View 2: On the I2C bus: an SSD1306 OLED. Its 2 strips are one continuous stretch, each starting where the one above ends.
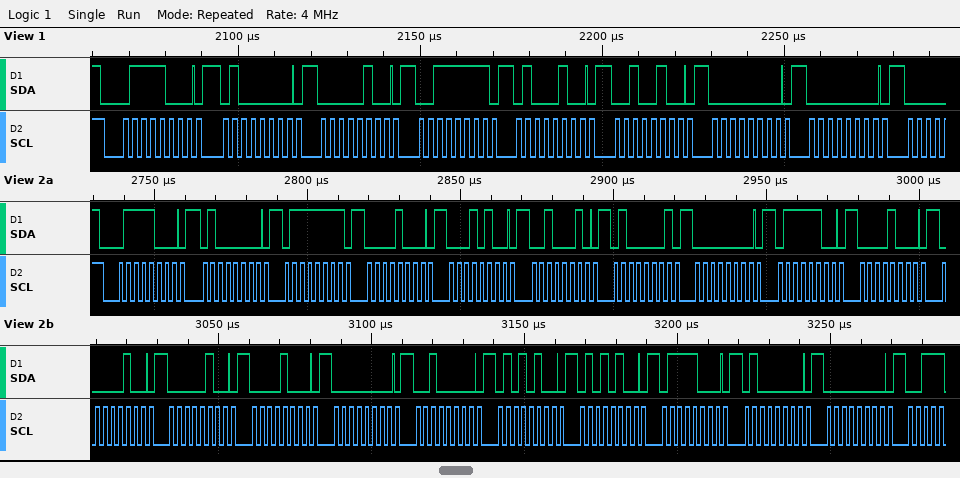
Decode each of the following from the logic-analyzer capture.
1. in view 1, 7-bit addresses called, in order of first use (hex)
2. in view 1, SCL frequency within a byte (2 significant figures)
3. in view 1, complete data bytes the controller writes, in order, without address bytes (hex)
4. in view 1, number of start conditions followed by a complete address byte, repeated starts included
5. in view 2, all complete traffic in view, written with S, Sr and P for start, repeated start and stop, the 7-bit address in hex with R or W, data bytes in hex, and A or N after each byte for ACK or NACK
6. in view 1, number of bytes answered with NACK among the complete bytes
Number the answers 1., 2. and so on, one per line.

1. 0x3C
2. 400 kHz
3. 40 04 3F 44 24 00 00
4. 1
5. S 3CW A 40 A 7F A 08 A 14 A 22 A 41 A 00 A 7C A 08 A 04 A 04 A 08 A 00 A 20 A 54 A 54 A 78 A 40 A 00 A
6. 0
